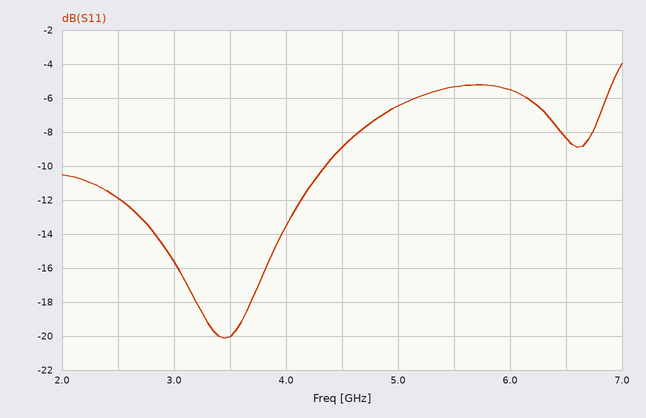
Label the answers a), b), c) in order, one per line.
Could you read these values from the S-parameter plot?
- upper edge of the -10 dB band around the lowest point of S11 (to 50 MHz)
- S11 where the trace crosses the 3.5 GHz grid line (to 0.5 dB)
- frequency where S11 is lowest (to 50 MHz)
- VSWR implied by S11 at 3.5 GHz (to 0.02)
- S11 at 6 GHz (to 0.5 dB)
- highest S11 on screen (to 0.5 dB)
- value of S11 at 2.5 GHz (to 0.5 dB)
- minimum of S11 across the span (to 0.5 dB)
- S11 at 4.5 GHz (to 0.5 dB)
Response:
a) 4.35 GHz
b) -20.0 dB
c) 3.45 GHz
d) 1.22
e) -5.5 dB
f) -4.0 dB
g) -12.0 dB
h) -20.0 dB
i) -9.0 dB
